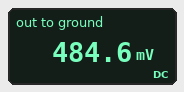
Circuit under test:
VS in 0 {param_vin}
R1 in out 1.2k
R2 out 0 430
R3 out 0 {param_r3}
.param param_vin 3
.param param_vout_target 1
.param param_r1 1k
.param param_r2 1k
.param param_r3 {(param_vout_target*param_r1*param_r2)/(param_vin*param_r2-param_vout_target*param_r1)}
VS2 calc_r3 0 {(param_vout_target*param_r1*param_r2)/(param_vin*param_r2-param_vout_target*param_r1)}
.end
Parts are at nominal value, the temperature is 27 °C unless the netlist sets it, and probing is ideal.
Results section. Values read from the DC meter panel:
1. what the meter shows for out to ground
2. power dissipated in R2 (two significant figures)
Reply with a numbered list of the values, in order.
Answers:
1. 484.6 mV
2. 550 µW
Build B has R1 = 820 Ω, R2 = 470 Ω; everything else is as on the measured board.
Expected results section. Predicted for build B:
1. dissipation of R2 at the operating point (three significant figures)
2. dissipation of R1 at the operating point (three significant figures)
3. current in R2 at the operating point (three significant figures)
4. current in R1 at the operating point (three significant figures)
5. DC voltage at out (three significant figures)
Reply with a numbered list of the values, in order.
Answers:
1. 996 µW
2. 6.54 mW
3. 1.46 mA
4. 2.82 mA
5. 684 mV
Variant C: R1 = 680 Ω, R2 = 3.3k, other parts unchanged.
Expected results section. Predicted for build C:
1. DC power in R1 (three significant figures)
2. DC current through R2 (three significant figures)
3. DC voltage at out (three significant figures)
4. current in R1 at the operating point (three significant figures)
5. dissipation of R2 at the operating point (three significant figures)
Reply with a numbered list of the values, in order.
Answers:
1. 4.93 mW
2. 354 µA
3. 1.17 V
4. 2.69 mA
5. 414 µW
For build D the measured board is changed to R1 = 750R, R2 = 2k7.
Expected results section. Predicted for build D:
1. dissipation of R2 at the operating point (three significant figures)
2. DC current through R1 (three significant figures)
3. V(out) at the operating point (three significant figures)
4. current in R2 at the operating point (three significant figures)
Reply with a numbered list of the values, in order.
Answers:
1. 432 µW
2. 2.56 mA
3. 1.08 V
4. 400 µA
